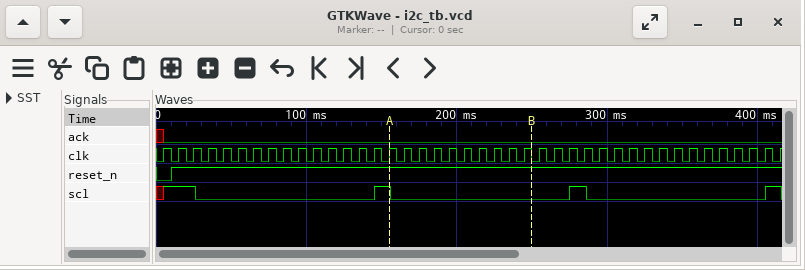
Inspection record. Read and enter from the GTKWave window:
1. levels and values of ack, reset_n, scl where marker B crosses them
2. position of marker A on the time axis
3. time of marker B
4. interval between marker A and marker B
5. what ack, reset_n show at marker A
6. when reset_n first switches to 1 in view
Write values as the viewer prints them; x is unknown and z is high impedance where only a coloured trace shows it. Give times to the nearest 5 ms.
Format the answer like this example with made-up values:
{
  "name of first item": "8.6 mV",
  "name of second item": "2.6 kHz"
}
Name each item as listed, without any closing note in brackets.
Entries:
{
  "levels and values of ack, reset_n, scl where marker B crosses them": "ack=0, reset_n=1, scl=0",
  "position of marker A on the time axis": "155 ms",
  "time of marker B": "250 ms",
  "interval between marker A and marker B": "95 ms",
  "what ack, reset_n show at marker A": "ack=0, reset_n=1",
  "when reset_n first switches to 1 in view": "10 ms"
}
